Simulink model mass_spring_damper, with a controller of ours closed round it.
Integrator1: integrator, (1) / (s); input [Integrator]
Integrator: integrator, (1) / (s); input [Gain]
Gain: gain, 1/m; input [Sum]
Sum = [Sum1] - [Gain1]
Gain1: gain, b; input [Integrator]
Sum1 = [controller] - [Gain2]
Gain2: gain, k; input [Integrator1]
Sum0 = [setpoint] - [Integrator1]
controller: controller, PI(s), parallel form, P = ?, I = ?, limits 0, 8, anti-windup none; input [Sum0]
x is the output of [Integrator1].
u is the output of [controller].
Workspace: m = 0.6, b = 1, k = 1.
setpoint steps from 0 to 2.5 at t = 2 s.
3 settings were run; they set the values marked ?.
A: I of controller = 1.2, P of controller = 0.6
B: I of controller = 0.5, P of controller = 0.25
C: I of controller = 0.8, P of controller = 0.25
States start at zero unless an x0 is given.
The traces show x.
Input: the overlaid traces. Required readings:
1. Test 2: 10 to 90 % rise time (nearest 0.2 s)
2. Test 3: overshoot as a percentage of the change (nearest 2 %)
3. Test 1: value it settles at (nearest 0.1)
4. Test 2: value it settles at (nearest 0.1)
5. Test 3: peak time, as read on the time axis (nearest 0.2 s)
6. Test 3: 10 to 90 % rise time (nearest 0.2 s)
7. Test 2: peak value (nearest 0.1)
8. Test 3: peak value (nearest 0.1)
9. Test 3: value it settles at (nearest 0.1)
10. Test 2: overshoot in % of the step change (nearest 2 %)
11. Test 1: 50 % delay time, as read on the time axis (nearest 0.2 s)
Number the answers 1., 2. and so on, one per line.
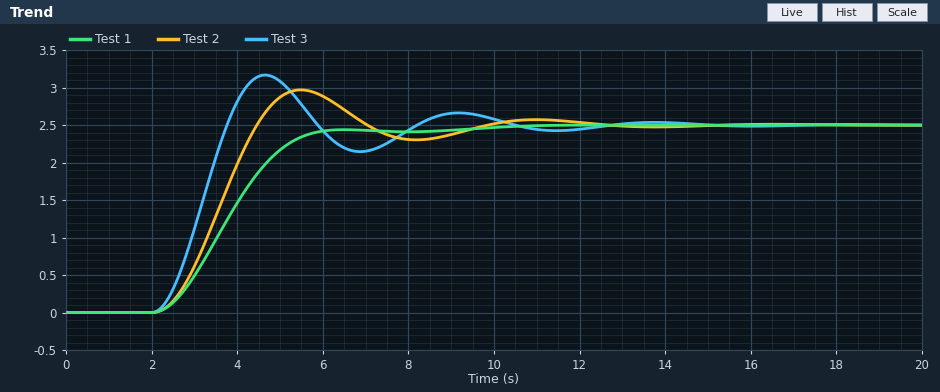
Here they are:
1. 1.6 s
2. 26 %
3. 2.5
4. 2.5
5. 4.6 s
6. 1.2 s
7. 3.0
8. 3.2
9. 2.5
10. 18 %
11. 3.8 s
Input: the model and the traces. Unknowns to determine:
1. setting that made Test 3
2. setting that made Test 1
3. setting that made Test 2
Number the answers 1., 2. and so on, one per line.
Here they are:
1. A
2. B
3. C
